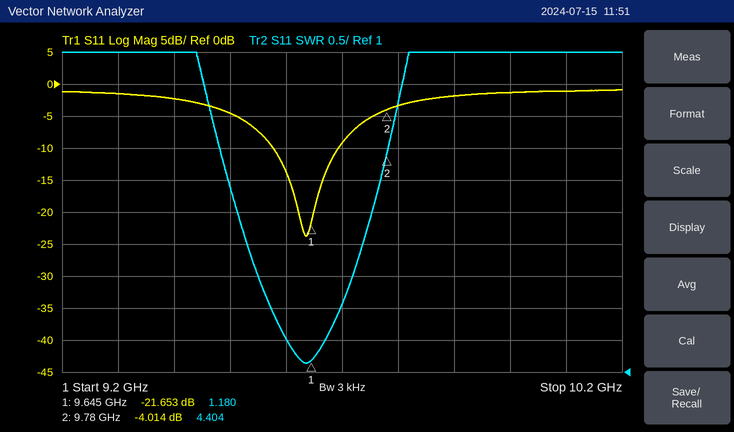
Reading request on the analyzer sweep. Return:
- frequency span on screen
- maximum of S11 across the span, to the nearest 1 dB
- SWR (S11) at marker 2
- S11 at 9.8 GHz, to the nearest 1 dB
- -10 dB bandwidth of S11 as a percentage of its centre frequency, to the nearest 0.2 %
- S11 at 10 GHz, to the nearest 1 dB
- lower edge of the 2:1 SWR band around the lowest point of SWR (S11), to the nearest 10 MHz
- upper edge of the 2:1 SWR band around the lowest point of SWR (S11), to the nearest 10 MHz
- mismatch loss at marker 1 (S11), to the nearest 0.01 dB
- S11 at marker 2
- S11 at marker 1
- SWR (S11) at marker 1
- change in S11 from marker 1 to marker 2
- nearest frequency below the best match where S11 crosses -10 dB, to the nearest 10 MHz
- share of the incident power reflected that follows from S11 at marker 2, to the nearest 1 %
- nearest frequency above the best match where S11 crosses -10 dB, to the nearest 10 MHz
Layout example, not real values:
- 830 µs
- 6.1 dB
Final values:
- 1 GHz
- -1 dB
- 4.404
- -3 dB
- 1.2 %
- -1 dB
- 9.57 GHz
- 9.70 GHz
- 0.03 dB
- -4.014 dB
- -21.653 dB
- 1.180
- 17.639 dB
- 9.58 GHz
- 40 %
- 9.69 GHz
